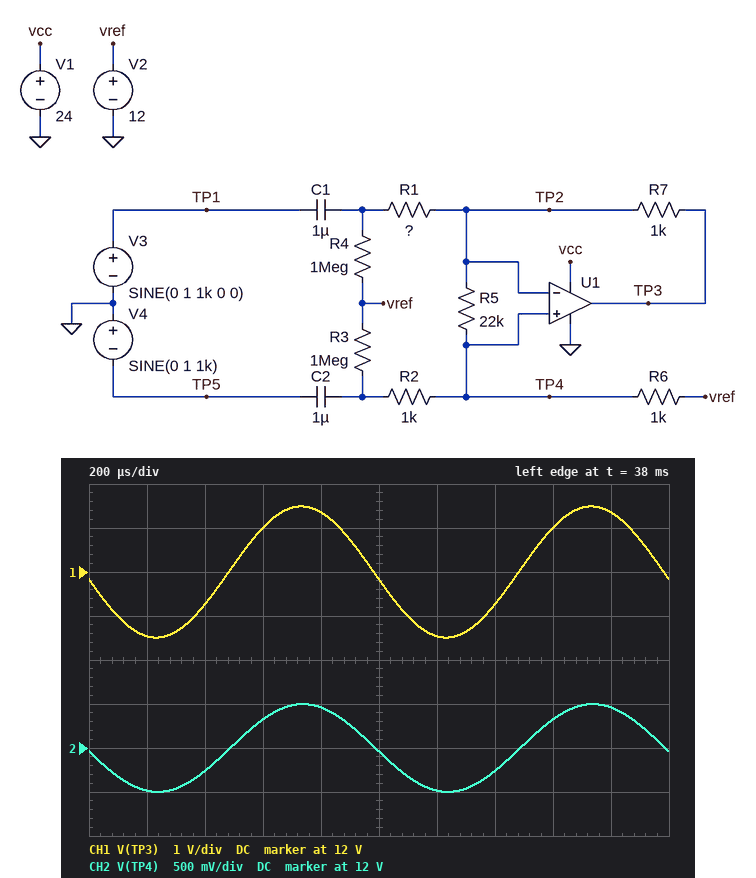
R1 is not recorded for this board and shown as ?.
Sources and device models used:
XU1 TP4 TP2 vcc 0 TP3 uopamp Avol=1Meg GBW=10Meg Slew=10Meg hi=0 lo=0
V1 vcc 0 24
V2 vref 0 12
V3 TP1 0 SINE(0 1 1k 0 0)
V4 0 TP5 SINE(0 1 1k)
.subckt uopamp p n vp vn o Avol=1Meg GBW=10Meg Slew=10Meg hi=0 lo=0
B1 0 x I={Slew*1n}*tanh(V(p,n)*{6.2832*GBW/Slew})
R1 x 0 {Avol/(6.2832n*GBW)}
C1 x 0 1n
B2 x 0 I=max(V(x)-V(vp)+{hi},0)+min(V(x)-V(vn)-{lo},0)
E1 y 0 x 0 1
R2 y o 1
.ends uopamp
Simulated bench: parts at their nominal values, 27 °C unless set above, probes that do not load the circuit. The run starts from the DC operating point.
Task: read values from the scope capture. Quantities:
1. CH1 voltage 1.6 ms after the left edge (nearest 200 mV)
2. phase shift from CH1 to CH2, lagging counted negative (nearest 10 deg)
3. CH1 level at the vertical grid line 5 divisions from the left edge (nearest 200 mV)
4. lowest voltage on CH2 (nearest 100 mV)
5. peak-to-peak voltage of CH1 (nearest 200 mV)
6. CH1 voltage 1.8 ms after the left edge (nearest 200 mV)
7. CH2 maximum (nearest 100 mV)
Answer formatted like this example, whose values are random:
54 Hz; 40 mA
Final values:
13.0 V; 0 deg; 11.8 V; 11.5 V; 3.0 V; 13.4 V; 12.5 V
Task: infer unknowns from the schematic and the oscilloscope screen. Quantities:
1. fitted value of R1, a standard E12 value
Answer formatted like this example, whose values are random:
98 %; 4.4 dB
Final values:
1.5 kΩ
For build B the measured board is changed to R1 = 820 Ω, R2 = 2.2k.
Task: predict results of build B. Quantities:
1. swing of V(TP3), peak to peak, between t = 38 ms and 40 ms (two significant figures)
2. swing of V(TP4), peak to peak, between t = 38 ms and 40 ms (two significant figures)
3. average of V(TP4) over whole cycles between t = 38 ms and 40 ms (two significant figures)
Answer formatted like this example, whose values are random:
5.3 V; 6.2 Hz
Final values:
3.8 V; 620 mV; 12 V
